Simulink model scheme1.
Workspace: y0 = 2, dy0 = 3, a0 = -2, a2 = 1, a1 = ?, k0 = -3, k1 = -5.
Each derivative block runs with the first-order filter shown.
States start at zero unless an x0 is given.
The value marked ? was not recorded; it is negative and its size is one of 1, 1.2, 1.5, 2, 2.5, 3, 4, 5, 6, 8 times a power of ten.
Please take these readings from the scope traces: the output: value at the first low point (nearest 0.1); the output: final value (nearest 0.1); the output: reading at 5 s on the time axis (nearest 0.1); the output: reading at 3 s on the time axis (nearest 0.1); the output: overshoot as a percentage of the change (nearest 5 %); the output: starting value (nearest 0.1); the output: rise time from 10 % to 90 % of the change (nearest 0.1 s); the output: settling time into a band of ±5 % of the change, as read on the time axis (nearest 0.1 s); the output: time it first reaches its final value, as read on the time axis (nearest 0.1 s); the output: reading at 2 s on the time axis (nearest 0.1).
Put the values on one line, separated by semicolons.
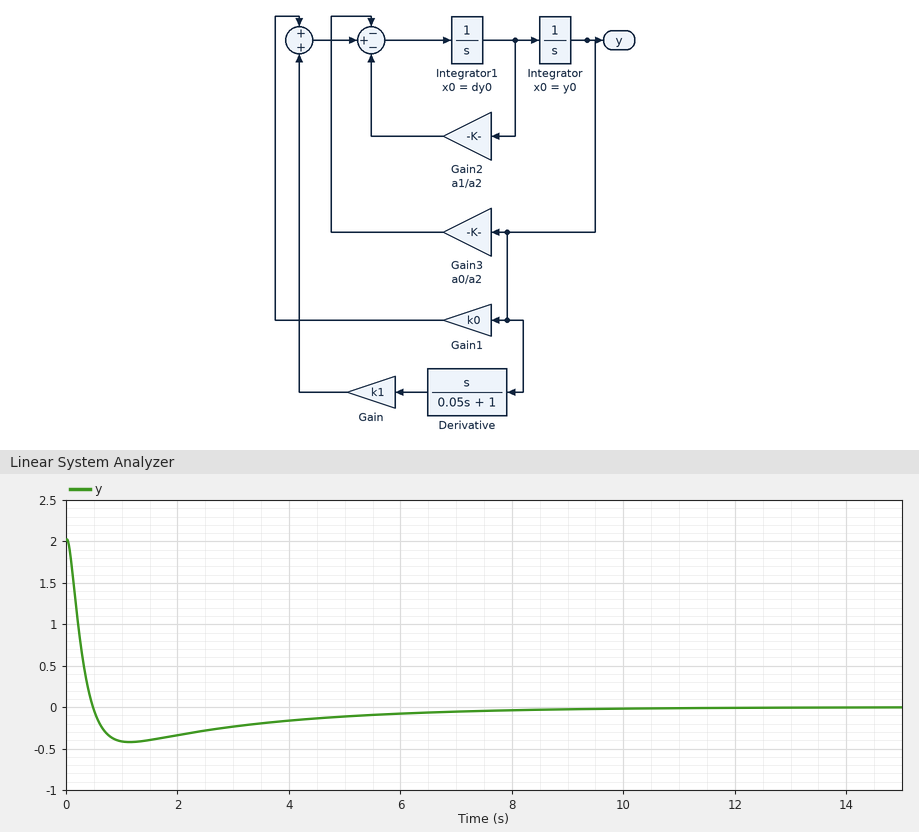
-0.4; 0.0; -0.1; -0.2; 20 %; 2.0; 0.3 s; 5.3 s; 0.5 s; -0.3
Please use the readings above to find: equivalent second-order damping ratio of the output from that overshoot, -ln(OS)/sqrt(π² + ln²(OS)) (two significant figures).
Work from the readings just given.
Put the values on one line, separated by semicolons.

0.46
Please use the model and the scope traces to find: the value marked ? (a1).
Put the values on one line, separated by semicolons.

-2
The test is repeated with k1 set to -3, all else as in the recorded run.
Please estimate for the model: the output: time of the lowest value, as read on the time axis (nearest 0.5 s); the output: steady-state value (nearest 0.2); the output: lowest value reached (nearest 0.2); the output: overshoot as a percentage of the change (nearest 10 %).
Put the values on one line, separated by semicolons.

2.0 s; 0.0; -1.0; 50 %
